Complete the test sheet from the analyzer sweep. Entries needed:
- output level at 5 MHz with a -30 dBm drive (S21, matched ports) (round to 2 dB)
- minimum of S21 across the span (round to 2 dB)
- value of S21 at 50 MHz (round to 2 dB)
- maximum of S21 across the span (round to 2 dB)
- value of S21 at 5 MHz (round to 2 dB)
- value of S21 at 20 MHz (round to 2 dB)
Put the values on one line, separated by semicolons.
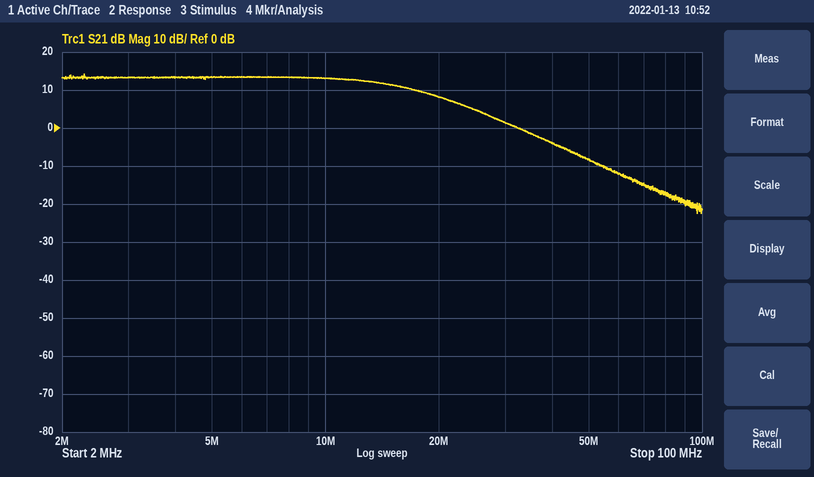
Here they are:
-16 dBm; -22 dB; -8 dB; 14 dB; 14 dB; 8 dB
